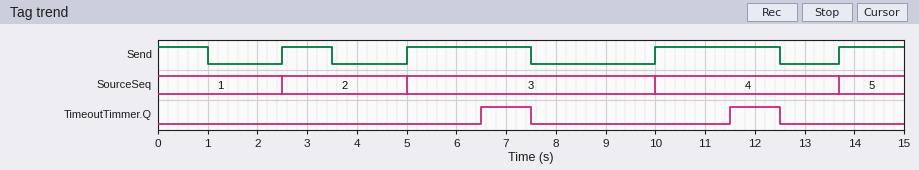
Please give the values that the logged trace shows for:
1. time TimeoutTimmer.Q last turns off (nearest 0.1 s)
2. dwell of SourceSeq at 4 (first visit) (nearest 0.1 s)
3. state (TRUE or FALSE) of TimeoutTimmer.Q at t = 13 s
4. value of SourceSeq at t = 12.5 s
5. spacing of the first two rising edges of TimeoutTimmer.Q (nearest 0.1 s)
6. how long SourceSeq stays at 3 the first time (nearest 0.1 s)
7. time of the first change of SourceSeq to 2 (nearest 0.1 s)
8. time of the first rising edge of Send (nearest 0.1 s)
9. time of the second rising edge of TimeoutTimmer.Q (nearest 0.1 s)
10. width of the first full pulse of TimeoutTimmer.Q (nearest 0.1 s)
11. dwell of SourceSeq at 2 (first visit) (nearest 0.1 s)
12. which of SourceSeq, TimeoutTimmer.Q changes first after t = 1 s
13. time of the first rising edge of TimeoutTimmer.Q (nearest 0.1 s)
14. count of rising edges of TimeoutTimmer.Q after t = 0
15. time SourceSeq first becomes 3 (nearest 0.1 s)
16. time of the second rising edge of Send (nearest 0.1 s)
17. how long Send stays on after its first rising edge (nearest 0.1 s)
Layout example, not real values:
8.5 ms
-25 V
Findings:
12.5 s
3.7 s
FALSE
4
5.0 s
5.0 s
2.5 s
2.5 s
11.5 s
1.0 s
2.5 s
SourceSeq
6.5 s
2
5.0 s
5.0 s
1.0 s
